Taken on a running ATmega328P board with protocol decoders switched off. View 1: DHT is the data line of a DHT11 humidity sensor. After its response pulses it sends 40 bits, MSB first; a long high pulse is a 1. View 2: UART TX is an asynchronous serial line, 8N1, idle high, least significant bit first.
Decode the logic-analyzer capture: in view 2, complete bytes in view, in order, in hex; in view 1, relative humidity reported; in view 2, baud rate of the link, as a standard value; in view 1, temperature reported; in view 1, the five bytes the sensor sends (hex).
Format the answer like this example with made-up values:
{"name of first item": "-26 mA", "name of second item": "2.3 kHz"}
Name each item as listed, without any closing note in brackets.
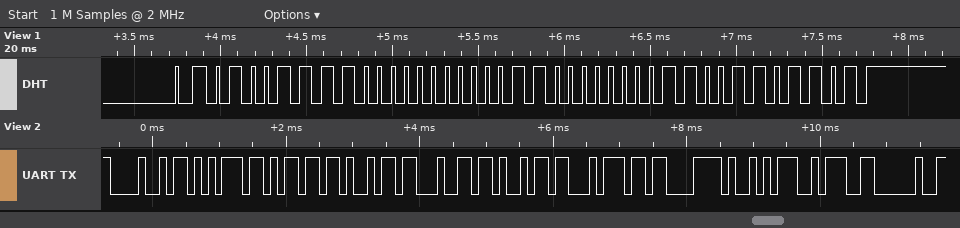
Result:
{"in view 2, complete bytes in view, in order, in hex": "48 75 6D 69 64 69 74 C3 A9 3A 20", "in view 1, relative humidity reported": "79 %", "in view 2, baud rate of the link, as a standard value": "9600 baud", "in view 1, temperature reported": "24.6 °C", "in view 1, the five bytes the sensor sends": "4F 00 18 06 6D"}
